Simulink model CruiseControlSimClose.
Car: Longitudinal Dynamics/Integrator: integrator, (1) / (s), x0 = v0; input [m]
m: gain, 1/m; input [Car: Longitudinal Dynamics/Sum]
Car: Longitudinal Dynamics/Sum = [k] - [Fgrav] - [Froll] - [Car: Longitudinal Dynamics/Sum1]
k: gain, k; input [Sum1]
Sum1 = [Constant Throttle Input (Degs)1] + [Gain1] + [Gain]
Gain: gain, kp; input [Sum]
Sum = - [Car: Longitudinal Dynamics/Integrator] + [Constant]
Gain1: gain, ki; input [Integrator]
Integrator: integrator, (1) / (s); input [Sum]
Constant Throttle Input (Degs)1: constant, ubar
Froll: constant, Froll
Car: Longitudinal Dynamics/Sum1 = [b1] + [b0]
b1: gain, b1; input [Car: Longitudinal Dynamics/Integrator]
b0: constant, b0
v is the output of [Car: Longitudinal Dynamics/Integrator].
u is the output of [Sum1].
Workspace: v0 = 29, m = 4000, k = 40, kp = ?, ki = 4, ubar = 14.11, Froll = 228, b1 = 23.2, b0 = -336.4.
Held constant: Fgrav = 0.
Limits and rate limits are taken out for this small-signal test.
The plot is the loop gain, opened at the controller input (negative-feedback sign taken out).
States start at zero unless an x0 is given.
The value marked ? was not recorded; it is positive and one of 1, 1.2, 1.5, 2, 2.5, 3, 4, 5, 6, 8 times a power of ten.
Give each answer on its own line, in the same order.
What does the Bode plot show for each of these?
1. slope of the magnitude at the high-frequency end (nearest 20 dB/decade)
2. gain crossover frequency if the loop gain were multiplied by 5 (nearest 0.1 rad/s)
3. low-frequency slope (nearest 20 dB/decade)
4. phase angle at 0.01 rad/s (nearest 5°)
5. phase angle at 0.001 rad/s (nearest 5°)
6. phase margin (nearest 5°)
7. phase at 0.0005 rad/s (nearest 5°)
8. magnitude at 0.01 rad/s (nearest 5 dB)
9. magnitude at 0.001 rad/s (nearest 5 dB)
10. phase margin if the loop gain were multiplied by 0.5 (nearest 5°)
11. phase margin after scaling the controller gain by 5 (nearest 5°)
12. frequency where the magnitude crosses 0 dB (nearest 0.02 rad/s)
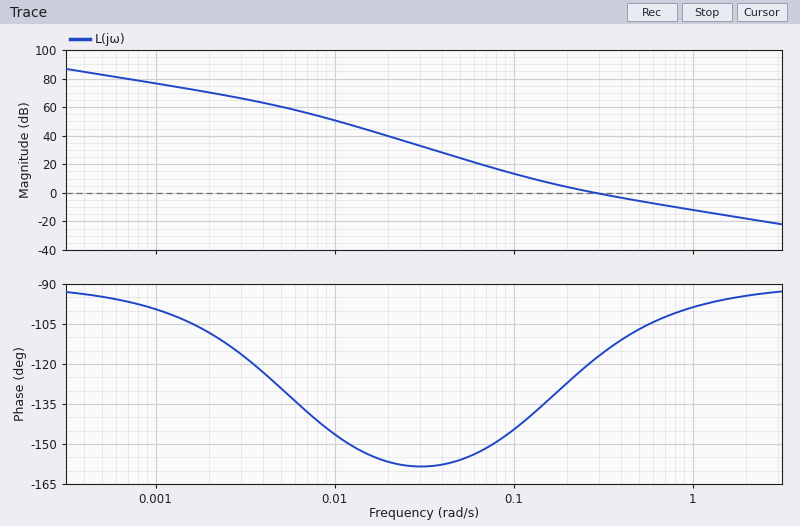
-20 dB/decade
1.3 rad/s
-20 dB/decade
-145°
-100°
60°
-95°
50 dB
75 dB
50°
85°
0.28 rad/s
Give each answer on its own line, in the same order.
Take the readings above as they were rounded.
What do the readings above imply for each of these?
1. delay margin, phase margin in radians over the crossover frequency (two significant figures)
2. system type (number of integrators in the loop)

3.7 s
1
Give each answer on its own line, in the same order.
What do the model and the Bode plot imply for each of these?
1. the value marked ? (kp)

25
